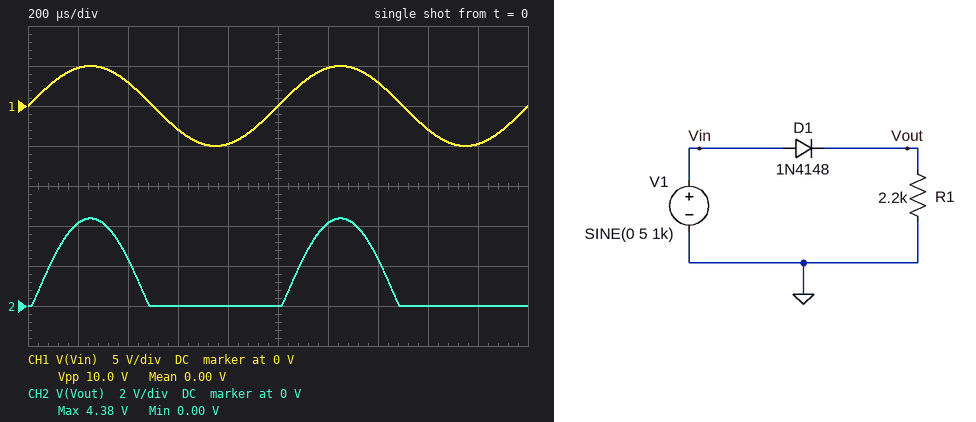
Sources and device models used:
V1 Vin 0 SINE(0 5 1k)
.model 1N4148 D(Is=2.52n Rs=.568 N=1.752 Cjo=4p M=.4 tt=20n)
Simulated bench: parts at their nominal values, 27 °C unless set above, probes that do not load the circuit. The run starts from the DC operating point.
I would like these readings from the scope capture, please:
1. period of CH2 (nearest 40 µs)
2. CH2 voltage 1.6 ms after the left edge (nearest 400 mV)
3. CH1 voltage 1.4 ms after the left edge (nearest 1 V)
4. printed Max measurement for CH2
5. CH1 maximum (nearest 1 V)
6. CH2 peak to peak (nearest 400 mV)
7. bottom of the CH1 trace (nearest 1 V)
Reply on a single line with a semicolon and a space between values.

1.00 ms; 0 V; 3 V; 4.38 V; 5 V; 4.4 V; -5 V
